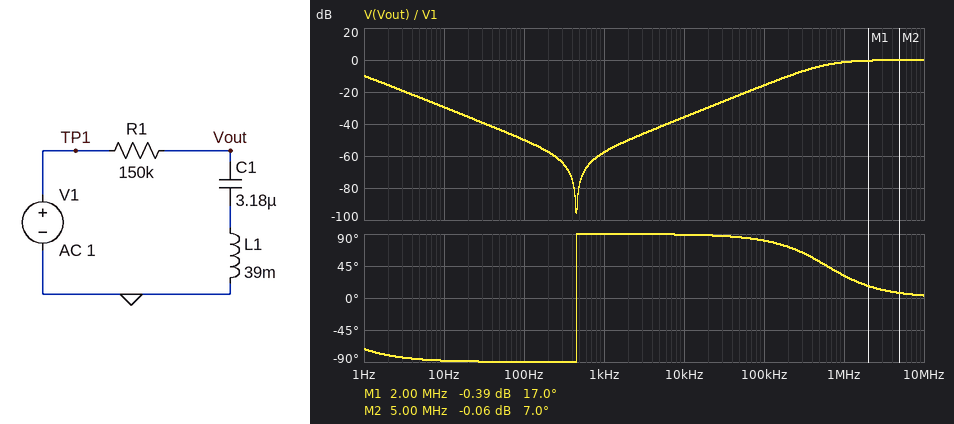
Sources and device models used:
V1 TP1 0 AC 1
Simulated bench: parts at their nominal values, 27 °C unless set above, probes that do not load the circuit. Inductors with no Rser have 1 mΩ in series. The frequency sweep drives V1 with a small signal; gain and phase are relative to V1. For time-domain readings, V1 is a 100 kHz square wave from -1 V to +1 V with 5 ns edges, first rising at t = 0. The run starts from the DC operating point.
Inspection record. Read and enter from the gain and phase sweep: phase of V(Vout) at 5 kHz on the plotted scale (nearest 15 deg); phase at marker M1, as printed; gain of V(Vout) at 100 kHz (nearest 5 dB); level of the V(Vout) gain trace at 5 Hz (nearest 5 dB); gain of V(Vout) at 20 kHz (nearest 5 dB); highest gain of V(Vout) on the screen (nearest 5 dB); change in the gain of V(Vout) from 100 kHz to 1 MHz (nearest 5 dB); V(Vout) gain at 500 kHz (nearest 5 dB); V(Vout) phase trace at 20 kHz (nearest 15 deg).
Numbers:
90 deg
17.0 deg
-15 dB
-25 dB
-30 dB
0 dB
15 dB
-5 dB
90 deg
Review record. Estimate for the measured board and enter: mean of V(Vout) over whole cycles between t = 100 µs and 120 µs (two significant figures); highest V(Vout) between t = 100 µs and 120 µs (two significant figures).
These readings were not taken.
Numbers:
-1.0 V
980 mV
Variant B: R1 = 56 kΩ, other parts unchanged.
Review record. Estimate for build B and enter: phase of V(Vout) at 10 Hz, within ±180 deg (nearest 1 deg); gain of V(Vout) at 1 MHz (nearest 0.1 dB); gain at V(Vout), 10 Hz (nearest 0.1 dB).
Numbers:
-85 deg
-0.2 dB
-21.0 dB
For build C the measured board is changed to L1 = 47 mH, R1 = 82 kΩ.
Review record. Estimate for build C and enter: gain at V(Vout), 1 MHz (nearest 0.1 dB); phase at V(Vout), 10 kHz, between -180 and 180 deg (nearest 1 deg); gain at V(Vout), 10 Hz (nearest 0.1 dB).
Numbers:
-0.3 dB
88 deg
-24.3 dB
